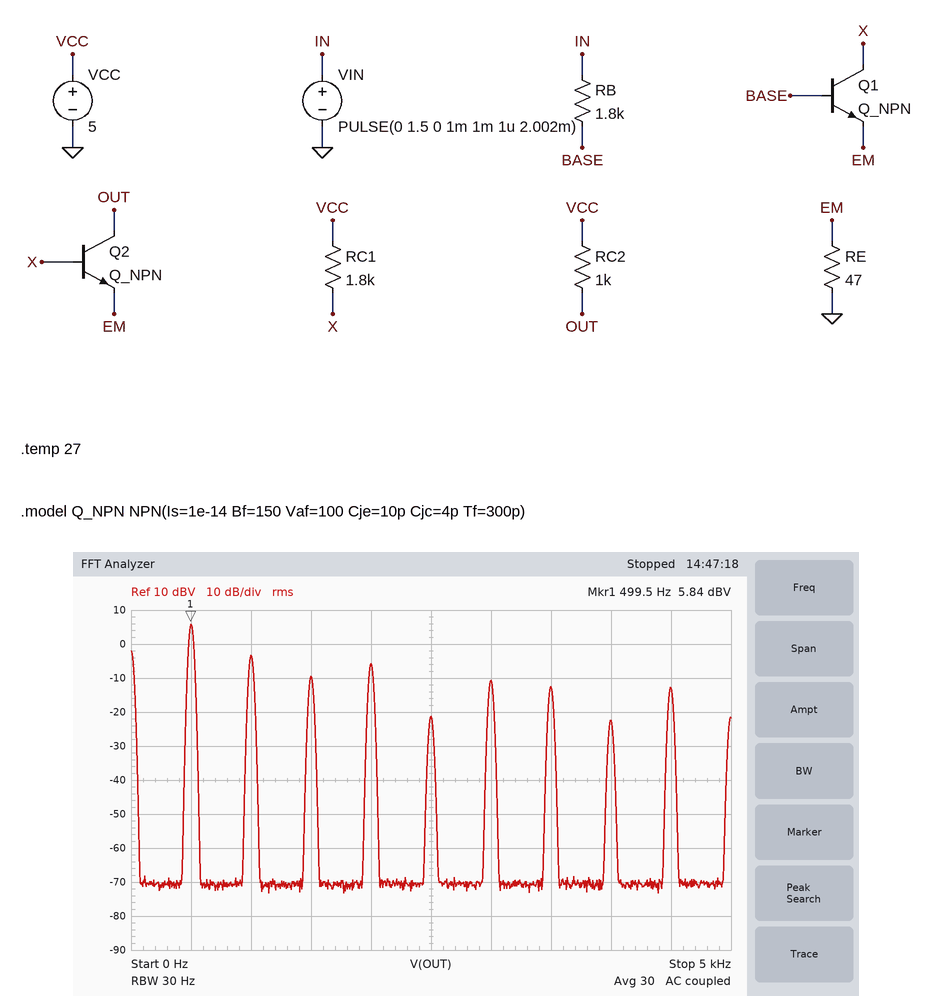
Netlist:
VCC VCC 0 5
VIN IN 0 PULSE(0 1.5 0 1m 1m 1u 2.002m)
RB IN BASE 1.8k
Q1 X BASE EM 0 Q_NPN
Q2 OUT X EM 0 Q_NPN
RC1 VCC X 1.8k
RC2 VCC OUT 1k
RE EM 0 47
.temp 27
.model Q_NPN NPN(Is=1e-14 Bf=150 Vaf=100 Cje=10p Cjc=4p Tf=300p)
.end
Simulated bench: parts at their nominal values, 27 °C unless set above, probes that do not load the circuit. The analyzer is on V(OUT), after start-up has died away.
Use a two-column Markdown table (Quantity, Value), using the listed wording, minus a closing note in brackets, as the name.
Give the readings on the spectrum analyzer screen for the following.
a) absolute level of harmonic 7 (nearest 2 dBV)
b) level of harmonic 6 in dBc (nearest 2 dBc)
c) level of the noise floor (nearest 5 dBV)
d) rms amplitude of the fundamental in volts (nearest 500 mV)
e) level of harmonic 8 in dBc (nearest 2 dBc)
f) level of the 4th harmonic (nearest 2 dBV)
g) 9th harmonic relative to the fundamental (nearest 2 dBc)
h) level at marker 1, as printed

| Quantity | Value |
|---|---|
| absolute level of harmonic 7 | -12 dBV |
| level of harmonic 6 in dBc | -16 dBc |
| level of the noise floor | -70 dBV |
| rms amplitude of the fundamental in volts | 2.0 V |
| level of harmonic 8 in dBc | -28 dBc |
| level of the 4th harmonic | -6 dBV |
| 9th harmonic relative to the fundamental | -18 dBc |
| level at marker 1, as printed | 5.84 dBV |
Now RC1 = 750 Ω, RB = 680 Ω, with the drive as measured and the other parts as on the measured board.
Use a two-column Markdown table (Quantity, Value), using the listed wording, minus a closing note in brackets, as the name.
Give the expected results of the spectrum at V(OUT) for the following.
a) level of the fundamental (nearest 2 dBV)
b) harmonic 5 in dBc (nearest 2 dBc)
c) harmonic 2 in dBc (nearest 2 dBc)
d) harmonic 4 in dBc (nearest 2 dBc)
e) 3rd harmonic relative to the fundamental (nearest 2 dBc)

| Quantity | Value |
|---|---|
| level of the fundamental | 4 dBV |
| harmonic 5 in dBc | -12 dBc |
| harmonic 2 in dBc | -4 dBc |
| harmonic 4 in dBc | -18 dBc |
| 3rd harmonic relative to the fundamental | -14 dBc |
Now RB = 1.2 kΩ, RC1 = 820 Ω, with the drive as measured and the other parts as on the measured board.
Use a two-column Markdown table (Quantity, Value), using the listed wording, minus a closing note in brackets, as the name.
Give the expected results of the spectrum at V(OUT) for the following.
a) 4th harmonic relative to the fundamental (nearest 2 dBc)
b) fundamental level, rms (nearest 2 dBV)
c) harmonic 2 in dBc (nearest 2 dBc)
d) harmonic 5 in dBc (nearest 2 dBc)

| Quantity | Value |
|---|---|
| 4th harmonic relative to the fundamental | -18 dBc |
| fundamental level, rms | 4 dBV |
| harmonic 2 in dBc | -4 dBc |
| harmonic 5 in dBc | -12 dBc |
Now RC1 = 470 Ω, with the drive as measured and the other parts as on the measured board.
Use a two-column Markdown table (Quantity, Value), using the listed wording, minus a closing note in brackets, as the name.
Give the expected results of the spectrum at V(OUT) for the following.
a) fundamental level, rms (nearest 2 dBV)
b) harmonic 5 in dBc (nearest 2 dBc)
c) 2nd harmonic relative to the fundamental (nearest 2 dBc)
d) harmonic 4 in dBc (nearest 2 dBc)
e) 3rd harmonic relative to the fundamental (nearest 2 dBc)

| Quantity | Value |
|---|---|
| fundamental level, rms | -2 dBV |
| harmonic 5 in dBc | -8 dBc |
| 2nd harmonic relative to the fundamental | 0 dBc |
| harmonic 4 in dBc | -4 dBc |
| 3rd harmonic relative to the fundamental | -2 dBc |
